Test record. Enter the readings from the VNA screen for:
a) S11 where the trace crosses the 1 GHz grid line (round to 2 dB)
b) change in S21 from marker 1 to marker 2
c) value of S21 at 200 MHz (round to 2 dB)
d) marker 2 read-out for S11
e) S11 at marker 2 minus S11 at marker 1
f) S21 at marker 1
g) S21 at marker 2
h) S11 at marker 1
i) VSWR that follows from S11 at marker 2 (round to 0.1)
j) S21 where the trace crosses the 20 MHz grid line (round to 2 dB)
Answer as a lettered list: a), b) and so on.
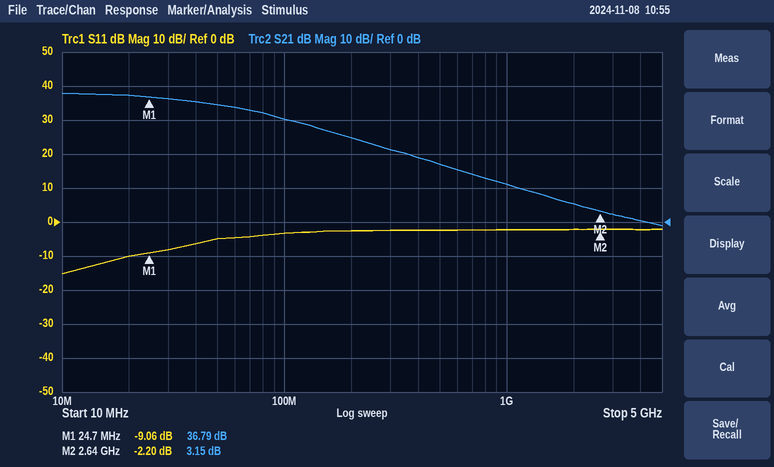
a) -2 dB
b) -33.64 dB
c) 24 dB
d) -2.20 dB
e) 6.86 dB
f) 36.79 dB
g) 3.15 dB
h) -9.06 dB
i) 7.9
j) 38 dB
